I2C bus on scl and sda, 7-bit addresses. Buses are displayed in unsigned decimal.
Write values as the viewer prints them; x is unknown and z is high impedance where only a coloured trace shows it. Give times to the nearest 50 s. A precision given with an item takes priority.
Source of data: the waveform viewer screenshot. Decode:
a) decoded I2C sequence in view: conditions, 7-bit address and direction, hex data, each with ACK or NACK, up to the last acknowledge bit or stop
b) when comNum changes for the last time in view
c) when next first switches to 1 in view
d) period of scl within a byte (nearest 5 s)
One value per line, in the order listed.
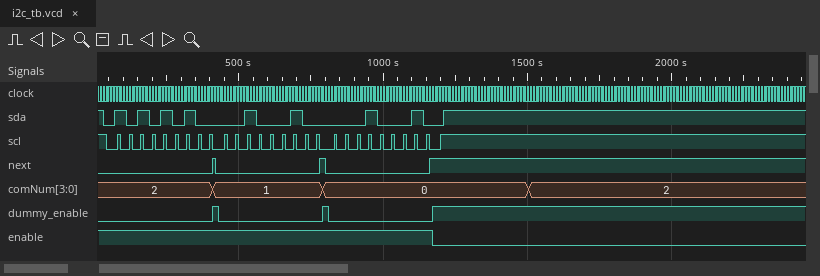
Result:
start, address 55 write ACK, 22 ACK, 11 ACK, stop
1500 s
400 s
40 s
